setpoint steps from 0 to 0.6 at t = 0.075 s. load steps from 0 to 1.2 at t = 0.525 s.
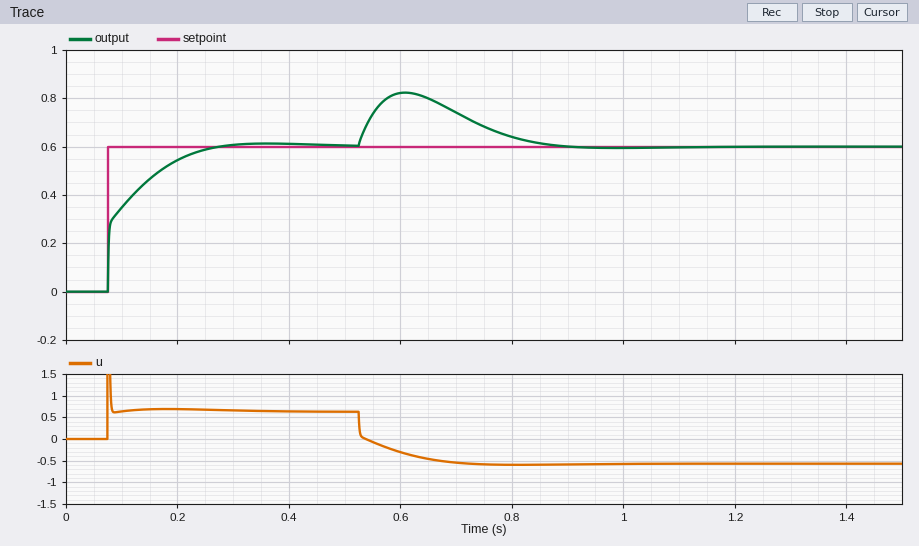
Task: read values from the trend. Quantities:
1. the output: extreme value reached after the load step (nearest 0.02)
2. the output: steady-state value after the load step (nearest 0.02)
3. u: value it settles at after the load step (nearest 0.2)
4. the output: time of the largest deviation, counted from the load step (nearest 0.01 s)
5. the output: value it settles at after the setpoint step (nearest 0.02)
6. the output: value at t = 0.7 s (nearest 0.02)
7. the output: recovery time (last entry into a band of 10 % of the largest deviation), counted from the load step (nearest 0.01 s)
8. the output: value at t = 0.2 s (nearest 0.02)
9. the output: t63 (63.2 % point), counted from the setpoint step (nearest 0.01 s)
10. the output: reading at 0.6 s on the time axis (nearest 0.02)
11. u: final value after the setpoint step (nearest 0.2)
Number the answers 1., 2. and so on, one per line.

1. 0.82
2. 0.60
3. -0.6
4. 0.08 s
5. 0.60
6. 0.74
7. 0.31 s
8. 0.54
9. 0.04 s
10. 0.82
11. 0.6
